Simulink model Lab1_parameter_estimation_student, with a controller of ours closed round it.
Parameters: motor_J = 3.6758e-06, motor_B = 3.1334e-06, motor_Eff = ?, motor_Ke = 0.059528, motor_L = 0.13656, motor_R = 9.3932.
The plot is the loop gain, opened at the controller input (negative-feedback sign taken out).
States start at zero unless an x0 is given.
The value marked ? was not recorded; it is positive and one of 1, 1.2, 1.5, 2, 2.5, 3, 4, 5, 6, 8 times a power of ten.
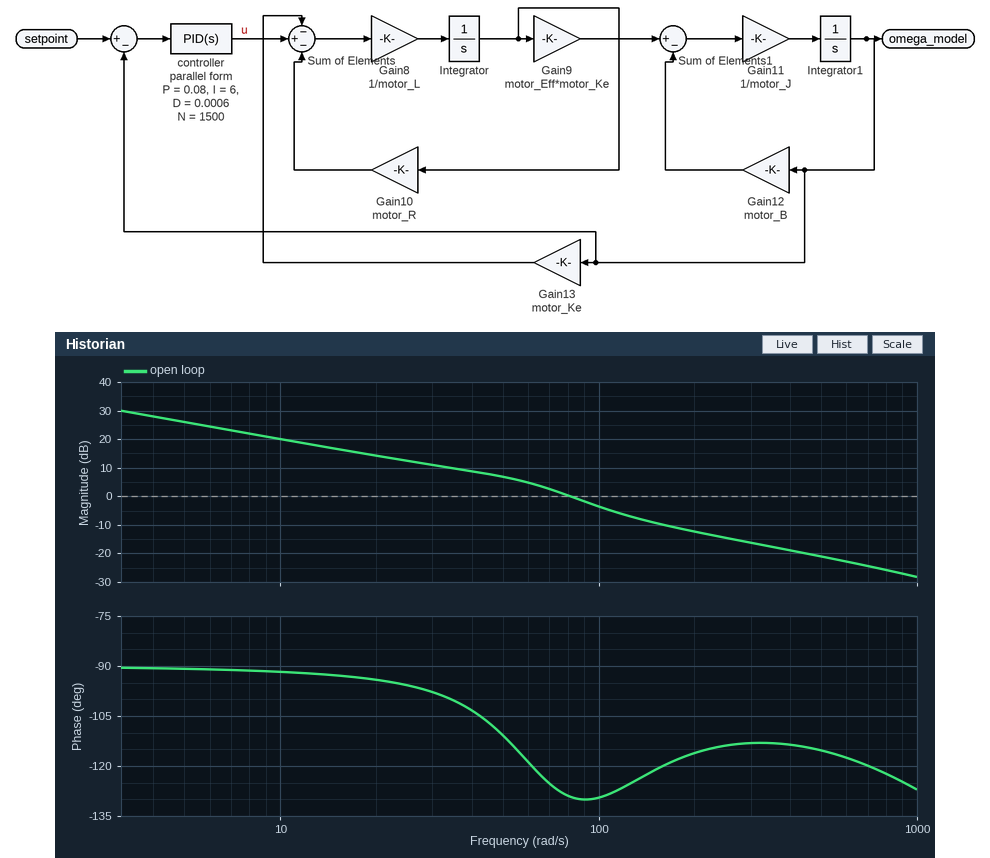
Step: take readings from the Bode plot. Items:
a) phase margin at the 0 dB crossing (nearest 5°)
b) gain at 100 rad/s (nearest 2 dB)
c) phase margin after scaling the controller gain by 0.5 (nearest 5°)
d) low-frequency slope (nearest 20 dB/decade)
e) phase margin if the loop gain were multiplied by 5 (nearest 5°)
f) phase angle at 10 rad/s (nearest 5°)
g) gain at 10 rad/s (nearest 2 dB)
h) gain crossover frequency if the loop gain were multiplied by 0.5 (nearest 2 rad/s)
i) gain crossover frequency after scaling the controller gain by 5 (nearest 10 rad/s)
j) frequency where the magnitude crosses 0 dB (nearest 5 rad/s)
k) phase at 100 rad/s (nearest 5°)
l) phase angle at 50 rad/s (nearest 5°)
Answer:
50°
-4 dB
65°
-20 dB/decade
65°
-90°
20 dB
54 rad/s
240 rad/s
80 rad/s
-130°
-110°
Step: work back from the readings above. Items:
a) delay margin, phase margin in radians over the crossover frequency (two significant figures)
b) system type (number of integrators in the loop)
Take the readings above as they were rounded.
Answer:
0.011 s
1
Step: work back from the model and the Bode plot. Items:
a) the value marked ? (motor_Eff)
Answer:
0.6
